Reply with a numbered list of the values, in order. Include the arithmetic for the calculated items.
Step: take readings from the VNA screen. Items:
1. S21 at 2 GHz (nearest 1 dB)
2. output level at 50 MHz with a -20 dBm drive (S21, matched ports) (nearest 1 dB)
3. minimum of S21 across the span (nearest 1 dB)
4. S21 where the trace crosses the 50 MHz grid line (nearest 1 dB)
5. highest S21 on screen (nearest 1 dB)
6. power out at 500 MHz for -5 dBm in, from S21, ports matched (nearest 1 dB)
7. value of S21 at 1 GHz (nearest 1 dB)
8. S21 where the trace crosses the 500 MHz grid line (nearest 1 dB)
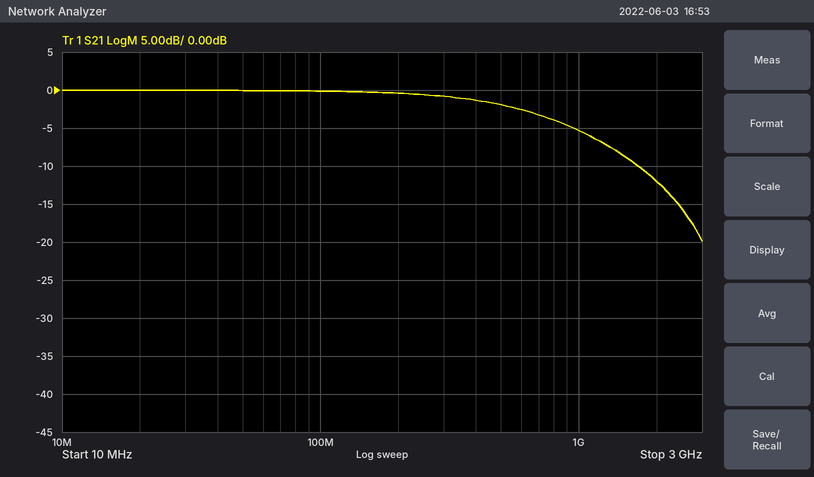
1. -12 dB
2. -20 dBm + (0 dB) = -20 dBm
3. -20 dB
4. 0 dB
5. 0 dB
6. -5 dBm + (-2 dB) = -7 dBm
7. -5 dB
8. -2 dB
